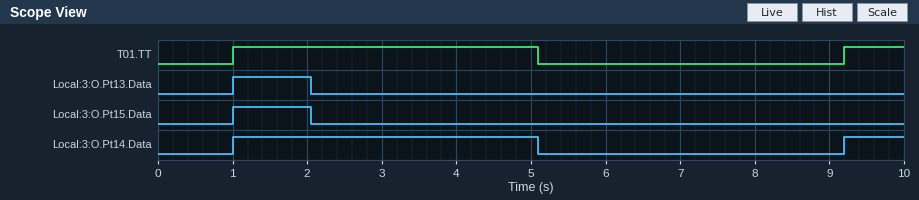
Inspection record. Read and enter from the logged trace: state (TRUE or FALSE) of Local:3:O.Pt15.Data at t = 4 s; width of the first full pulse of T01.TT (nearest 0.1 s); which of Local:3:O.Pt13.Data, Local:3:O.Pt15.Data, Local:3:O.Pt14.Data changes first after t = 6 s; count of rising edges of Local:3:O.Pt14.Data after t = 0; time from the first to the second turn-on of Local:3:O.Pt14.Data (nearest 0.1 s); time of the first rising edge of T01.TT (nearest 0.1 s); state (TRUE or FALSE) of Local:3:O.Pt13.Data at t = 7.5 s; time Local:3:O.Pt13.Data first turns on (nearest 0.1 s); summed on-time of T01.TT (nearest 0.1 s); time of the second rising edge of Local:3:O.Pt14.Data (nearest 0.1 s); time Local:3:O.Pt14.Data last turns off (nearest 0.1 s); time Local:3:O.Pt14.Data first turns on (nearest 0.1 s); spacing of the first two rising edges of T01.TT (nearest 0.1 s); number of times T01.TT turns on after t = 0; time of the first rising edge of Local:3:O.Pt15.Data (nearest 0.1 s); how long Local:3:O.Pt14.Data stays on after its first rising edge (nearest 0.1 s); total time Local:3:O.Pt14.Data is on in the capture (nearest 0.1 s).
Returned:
FALSE
4.1 s
Local:3:O.Pt14.Data
2
8.2 s
1.0 s
FALSE
1.0 s
4.9 s
9.2 s
5.1 s
1.0 s
8.2 s
2
1.0 s
4.1 s
4.9 s
